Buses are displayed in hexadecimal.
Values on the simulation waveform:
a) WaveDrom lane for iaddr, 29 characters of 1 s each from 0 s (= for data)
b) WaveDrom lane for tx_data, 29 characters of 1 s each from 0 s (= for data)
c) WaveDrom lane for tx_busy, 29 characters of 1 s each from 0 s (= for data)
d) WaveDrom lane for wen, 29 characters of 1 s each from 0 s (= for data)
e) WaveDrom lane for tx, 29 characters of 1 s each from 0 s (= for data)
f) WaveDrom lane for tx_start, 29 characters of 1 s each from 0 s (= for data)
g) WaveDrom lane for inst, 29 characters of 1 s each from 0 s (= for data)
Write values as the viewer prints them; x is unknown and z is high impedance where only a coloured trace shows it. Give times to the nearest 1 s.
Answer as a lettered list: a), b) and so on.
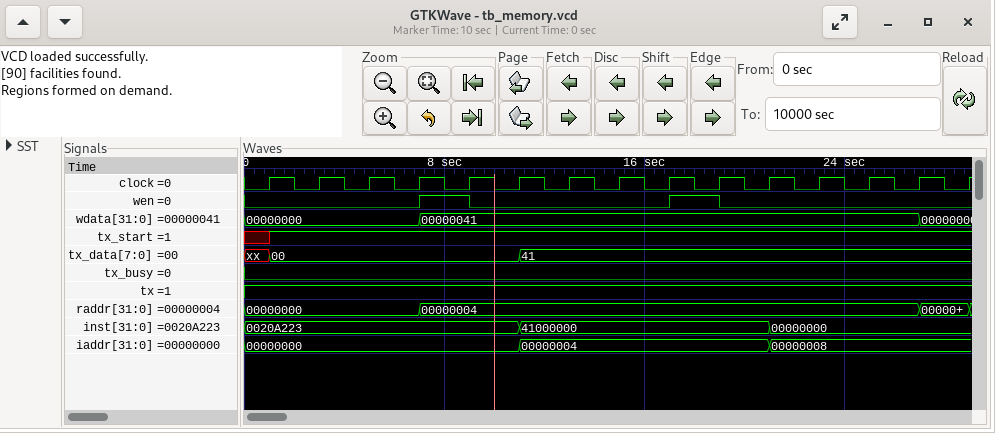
a) {name: 'iaddr', wave: '=..........=.........=.......', data: '00000000 00000004 00000008'}
b) {name: 'tx_data', wave: 'x=.........=.................', data: '00 41'}
c) {name: 'tx_busy', wave: '0............................'}
d) {name: 'wen', wave: '0......1.0.......1.0.........'}
e) {name: 'tx', wave: '1............................'}
f) {name: 'tx_start', wave: 'x1...........................'}
g) {name: 'inst', wave: '=..........=.........=.......', data: '0020A223 41000000 00000000'}
